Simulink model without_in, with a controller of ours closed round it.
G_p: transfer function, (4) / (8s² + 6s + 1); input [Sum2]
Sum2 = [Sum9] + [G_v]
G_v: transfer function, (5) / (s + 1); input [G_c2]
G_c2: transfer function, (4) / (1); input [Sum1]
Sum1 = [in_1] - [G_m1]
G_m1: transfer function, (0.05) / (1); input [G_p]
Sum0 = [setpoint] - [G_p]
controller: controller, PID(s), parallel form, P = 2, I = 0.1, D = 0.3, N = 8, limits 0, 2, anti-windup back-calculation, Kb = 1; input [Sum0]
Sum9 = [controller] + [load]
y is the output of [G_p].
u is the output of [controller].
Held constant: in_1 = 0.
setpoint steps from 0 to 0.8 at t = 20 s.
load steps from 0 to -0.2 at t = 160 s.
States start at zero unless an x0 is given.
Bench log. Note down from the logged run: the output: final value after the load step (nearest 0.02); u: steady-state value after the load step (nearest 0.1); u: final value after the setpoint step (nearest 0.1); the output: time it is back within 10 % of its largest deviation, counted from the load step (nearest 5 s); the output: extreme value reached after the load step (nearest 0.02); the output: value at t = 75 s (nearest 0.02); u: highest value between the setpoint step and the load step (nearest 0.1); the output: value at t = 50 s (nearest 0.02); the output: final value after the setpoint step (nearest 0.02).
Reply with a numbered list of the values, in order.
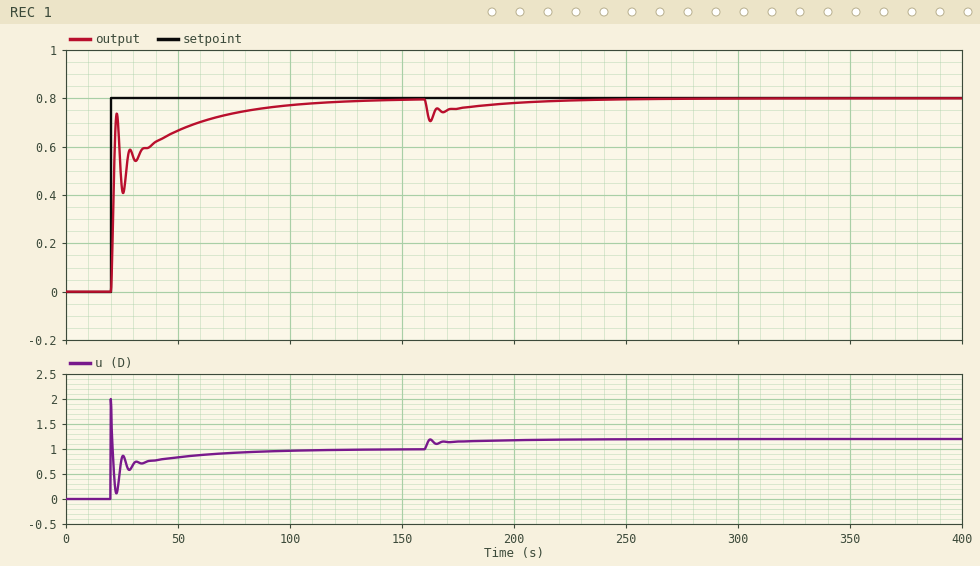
1. 0.80
2. 1.2
3. 1.0
4. 65 s
5. 0.70
6. 0.74
7. 2.0
8. 0.66
9. 0.80
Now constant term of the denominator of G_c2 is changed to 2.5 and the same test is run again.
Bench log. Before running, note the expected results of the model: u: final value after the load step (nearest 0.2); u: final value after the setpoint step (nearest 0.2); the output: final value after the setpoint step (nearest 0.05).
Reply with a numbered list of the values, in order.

1. 0.8
2. 0.6
3. 0.80
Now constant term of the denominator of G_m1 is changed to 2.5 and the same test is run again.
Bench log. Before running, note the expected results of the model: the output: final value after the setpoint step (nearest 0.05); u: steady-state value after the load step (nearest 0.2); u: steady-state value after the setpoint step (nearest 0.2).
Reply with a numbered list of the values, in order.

1. 0.80
2. 0.8
3. 0.6
